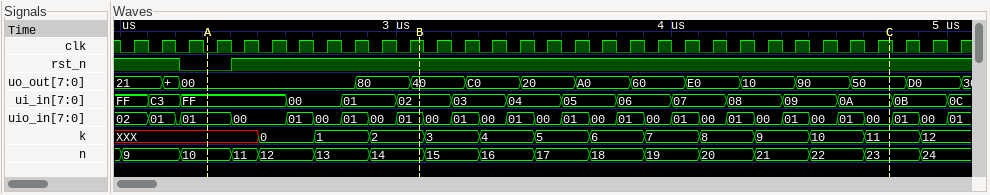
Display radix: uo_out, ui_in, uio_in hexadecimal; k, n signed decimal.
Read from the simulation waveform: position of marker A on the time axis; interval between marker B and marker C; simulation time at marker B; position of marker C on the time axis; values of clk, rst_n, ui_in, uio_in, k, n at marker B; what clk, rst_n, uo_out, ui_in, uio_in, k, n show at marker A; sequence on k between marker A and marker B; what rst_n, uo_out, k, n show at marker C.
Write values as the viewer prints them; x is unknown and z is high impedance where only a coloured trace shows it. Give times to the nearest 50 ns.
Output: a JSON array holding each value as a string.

["2300 ns", "1700 ns", "3100 ns", "4800 ns", "clk=1, rst_n=1, ui_in=02, uio_in=01, k=2, n=14", "clk=0, rst_n=0, uo_out=00, ui_in=FF, uio_in=01, k=XXX, n=10", "XXX, 0, 1, 2", "rst_n=1, uo_out=50, k=11, n=23"]
